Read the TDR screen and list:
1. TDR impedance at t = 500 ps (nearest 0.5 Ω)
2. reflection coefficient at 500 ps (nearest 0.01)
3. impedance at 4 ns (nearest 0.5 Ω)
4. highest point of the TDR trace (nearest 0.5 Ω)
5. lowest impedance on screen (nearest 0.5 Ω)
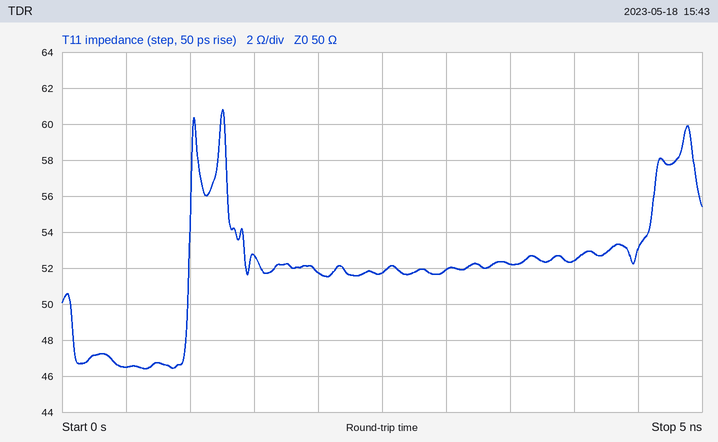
46.5 Ω
-0.04
52.5 Ω
61.0 Ω
46.5 Ω
